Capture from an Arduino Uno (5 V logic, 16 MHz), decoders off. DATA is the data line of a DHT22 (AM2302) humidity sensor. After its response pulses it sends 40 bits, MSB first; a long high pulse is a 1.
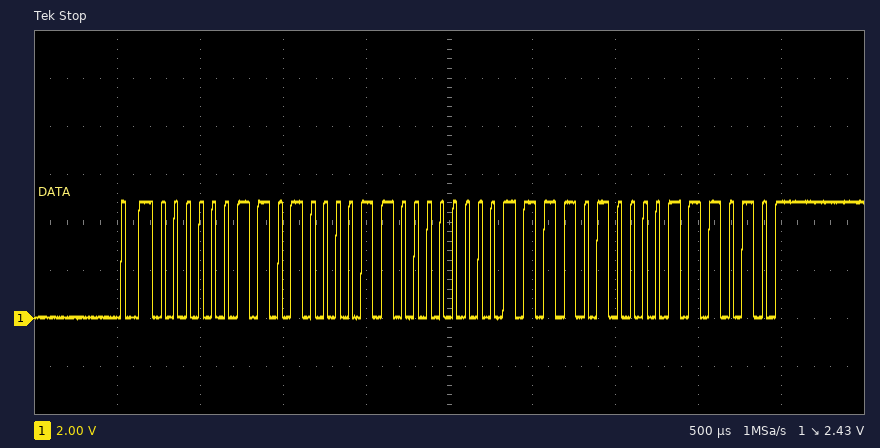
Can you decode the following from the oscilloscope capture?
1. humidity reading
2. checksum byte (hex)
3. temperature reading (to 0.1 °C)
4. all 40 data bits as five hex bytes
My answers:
83.5 %
0x3A
24.4 °C
03 43 00 F4 3A
